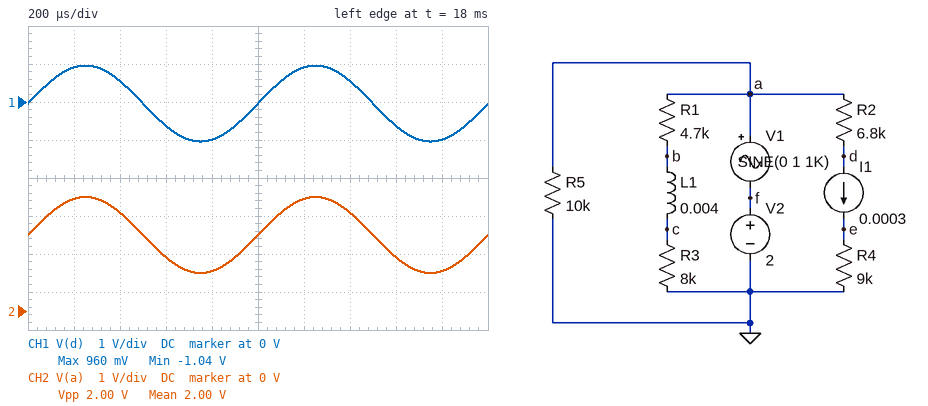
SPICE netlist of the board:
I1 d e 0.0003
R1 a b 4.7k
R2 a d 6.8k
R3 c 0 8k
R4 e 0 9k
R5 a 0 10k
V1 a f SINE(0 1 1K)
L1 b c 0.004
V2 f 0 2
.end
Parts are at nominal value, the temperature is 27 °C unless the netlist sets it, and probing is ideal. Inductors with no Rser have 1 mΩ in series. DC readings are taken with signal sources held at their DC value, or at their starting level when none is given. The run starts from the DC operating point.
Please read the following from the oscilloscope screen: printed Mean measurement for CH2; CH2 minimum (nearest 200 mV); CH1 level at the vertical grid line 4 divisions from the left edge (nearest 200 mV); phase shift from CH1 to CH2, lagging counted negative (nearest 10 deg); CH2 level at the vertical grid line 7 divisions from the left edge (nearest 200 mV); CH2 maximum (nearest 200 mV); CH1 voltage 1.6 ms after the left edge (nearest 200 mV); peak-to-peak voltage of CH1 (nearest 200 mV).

2.00 V
1.0 V
-1.0 V
0 deg
2.6 V
3.0 V
-600 mV
2.0 V
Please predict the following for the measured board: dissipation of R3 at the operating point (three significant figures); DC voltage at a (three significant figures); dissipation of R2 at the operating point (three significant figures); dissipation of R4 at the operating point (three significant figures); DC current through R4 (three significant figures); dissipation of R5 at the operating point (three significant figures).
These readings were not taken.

198 µW
2.00 V
612 µW
810 µW
300 µA
400 µW
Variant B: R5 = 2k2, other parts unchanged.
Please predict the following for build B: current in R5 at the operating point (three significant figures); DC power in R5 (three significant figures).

909 µA
1.82 mW
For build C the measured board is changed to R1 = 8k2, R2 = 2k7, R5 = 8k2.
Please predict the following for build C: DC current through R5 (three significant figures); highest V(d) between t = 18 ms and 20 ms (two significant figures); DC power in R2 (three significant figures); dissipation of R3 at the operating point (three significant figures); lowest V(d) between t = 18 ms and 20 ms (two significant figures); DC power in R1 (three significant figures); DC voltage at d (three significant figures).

244 µA
2.2 V
243 µW
122 µW
190 mV
125 µW
1.19 V
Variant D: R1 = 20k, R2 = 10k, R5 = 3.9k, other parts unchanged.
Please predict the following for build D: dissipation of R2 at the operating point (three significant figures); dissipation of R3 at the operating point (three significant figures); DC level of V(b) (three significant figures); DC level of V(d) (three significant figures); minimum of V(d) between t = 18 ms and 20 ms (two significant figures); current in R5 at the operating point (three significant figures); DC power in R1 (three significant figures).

900 µW
40.8 µW
571 mV
-1.00 V
-2.0 V
513 µA
102 µW
